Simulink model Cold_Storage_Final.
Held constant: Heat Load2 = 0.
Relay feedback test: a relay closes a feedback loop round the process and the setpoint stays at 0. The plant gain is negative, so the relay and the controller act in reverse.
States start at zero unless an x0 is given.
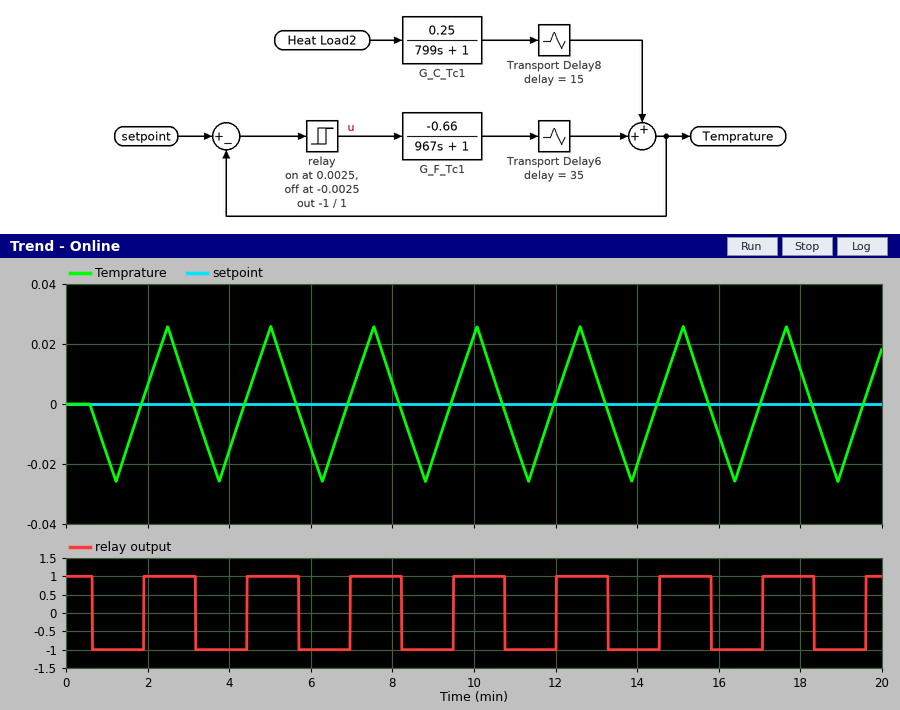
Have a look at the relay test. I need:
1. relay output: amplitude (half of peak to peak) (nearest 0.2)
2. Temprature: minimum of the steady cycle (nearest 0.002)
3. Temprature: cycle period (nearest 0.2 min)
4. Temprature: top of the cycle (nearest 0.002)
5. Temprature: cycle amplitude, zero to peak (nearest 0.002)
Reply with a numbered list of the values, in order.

1. 1.0
2. -0.026
3. 2.6 min
4. 0.026
5. 0.026
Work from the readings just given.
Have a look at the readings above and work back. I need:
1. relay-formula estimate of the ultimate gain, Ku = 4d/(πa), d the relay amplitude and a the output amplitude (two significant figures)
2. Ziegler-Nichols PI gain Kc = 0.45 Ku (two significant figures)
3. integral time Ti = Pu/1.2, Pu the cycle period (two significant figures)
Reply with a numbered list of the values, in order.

1. 49
2. 22
3. 2.2 min
